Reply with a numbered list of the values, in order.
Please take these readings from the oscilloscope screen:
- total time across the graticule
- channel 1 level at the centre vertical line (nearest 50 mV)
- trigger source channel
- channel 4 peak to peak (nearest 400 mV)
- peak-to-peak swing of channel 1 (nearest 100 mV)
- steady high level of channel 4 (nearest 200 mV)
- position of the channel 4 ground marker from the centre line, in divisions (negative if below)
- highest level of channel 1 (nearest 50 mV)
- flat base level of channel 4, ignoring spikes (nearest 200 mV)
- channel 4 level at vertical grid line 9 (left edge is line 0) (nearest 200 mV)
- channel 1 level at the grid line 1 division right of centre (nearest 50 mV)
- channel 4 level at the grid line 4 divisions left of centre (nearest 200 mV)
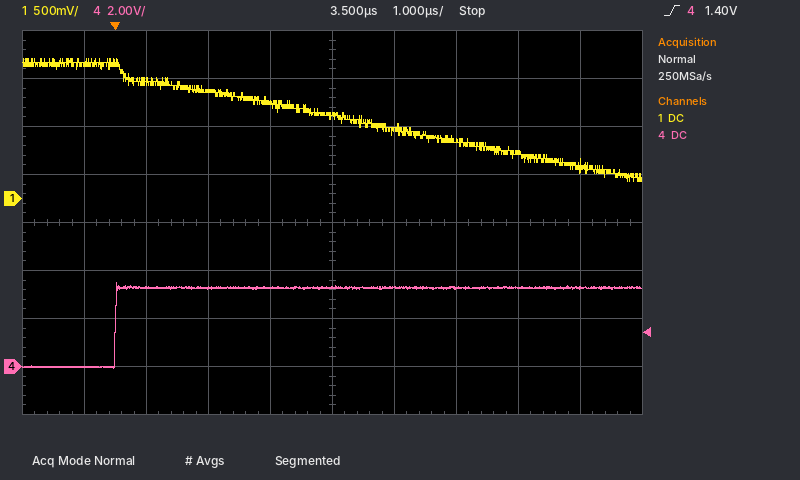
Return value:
1. 10 µs
2. 850 mV
3. channel 4
4. 3.6 V
5. 1.30 V
6. 3.2 V
7. -3.0 div
8. 1.45 V
9. 0.0 V
10. 3.2 V
11. 700 mV
12. 0.0 V
